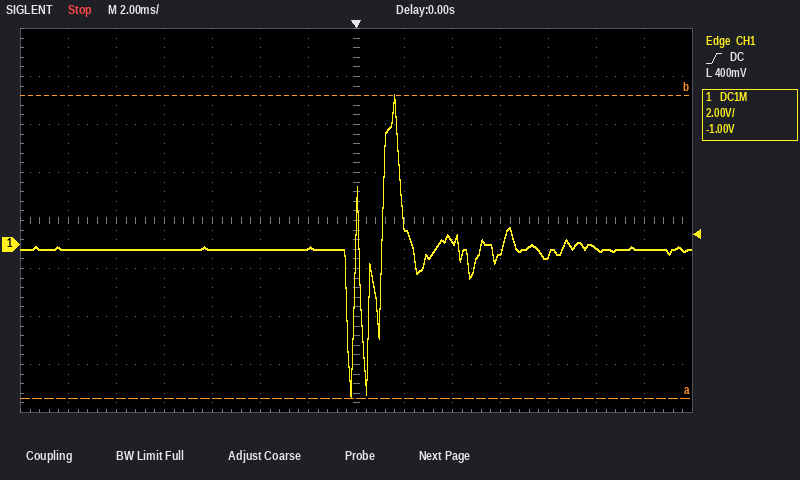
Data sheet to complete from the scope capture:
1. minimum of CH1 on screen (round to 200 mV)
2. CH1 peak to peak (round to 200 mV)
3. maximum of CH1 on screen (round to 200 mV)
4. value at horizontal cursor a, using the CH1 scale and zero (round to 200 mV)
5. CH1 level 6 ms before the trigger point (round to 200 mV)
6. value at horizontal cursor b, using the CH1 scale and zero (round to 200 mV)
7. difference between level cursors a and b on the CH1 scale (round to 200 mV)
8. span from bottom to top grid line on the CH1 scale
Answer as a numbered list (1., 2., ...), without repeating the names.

1. -6.4 V
2. 12.6 V
3. 6.2 V
4. -6.4 V
5. -200 mV
6. 6.2 V
7. 12.6 V
8. 16 V
